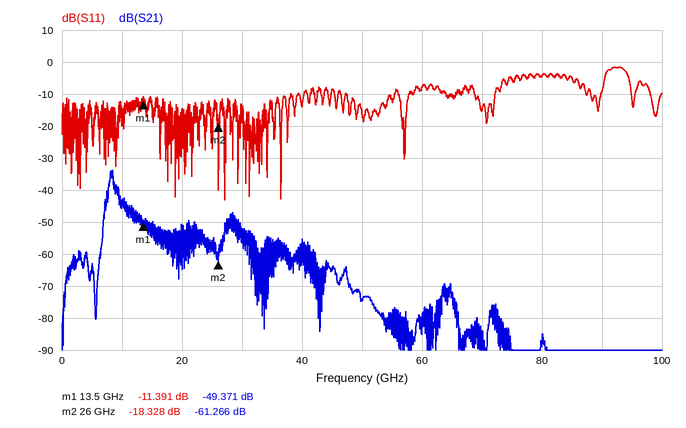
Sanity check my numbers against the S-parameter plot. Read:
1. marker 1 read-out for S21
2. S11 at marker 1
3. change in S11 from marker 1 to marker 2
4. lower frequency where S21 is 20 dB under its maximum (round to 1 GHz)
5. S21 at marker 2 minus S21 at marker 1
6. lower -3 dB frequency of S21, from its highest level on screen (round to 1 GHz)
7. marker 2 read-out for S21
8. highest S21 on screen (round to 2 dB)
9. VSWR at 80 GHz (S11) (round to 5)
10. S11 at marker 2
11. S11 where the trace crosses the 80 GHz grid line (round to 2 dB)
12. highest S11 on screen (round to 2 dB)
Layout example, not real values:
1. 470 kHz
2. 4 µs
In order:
1. -49.371 dB
2. -11.391 dB
3. -6.937 dB
4. 7 GHz
5. -11.895 dB
6. 8 GHz
7. -61.266 dB
8. -34 dB
9. 5
10. -18.328 dB
11. -4 dB
12. -2 dB
